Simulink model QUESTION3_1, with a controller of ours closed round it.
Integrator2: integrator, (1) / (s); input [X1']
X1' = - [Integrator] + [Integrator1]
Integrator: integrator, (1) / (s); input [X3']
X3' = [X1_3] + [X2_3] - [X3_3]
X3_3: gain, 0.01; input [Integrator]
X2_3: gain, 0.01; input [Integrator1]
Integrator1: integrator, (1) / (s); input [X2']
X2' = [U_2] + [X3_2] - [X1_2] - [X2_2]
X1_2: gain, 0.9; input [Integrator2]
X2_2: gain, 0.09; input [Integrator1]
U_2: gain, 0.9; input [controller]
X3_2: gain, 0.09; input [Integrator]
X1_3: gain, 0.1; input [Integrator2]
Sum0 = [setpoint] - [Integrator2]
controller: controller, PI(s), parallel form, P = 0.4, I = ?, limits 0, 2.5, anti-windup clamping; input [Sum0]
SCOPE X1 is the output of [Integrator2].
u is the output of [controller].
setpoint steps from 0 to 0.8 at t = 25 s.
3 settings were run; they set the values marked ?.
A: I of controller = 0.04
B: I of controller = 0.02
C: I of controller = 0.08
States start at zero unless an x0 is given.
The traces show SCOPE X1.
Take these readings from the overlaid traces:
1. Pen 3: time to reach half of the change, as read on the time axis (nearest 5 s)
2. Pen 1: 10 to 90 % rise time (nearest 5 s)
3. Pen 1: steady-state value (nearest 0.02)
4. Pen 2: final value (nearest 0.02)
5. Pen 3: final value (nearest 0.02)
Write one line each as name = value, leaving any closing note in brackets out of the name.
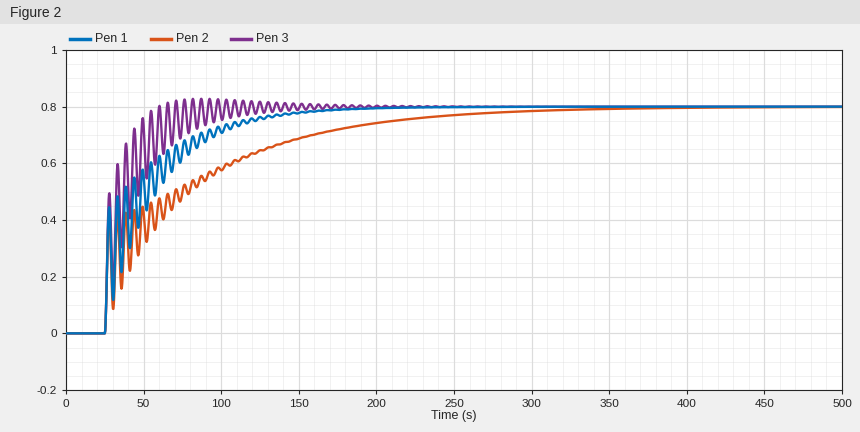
Pen 3: time to reach half of the change, as read on the time axis = 25 s
Pen 1: 10 to 90 % rise time = 70 s
Pen 1: steady-state value = 0.80
Pen 2: final value = 0.80
Pen 3: final value = 0.80
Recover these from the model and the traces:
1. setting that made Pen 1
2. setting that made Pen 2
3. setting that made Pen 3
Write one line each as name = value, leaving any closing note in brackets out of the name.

setting that made Pen 1 = A
setting that made Pen 2 = B
setting that made Pen 3 = C
